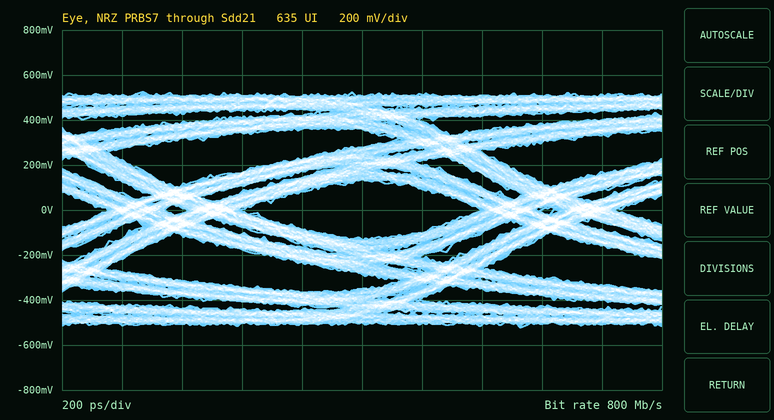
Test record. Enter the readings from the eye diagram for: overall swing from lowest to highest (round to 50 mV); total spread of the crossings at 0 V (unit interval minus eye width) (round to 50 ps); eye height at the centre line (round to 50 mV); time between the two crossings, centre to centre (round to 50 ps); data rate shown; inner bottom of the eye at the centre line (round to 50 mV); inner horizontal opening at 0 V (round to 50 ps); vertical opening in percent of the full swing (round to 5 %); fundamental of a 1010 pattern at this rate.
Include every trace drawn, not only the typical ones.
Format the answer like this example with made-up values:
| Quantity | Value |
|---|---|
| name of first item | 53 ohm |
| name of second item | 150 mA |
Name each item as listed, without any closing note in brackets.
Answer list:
| Quantity | Value |
|---|---|
| overall swing from lowest to highest | 1.05 V |
| total spread of the crossings at 0 V (unit interval minus eye width) | 450 ps |
| eye height at the centre line | 250 mV |
| time between the two crossings, centre to centre | 1.25 ns |
| data rate shown | 800 Mb/s |
| inner bottom of the eye at the centre line | -150 mV |
| inner horizontal opening at 0 V | 800 ps |
| vertical opening in percent of the full swing | 25 % |
| fundamental of a 1010 pattern at this rate | 400 MHz |
